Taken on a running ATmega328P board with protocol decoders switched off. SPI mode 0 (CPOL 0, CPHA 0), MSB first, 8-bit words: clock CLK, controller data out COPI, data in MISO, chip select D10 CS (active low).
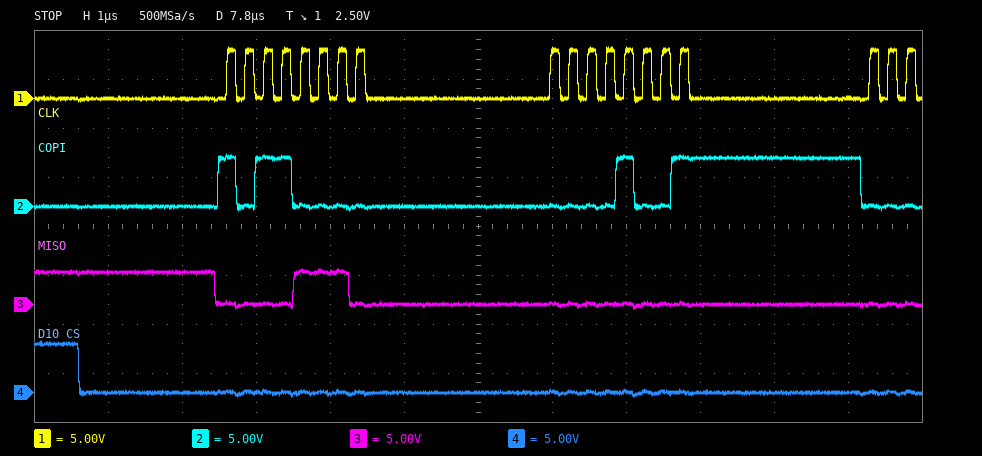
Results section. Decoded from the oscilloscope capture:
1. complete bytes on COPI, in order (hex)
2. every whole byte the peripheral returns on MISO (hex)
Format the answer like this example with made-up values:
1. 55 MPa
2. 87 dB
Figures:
1. B0 09
2. 0E 00
